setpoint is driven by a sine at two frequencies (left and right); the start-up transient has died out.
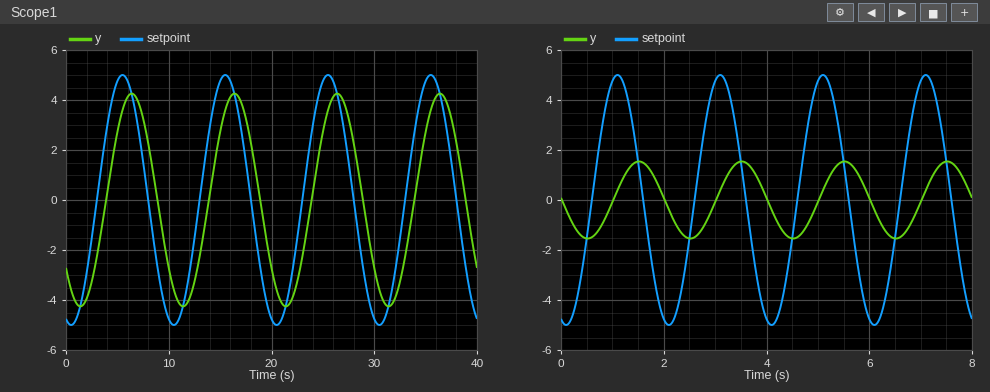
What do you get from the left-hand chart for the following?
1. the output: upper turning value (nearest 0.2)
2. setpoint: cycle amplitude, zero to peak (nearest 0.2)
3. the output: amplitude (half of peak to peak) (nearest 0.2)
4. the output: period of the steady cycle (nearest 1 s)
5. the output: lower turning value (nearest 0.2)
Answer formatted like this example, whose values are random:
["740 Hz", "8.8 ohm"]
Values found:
["4.2", "5.0", "4.2", "10 s", "-4.2"]
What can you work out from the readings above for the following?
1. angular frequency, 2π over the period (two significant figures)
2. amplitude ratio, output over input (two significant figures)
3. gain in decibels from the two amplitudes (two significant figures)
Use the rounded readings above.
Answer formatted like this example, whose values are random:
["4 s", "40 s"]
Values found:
["0.63 rad/s", "0.84", "-1.5 dB"]
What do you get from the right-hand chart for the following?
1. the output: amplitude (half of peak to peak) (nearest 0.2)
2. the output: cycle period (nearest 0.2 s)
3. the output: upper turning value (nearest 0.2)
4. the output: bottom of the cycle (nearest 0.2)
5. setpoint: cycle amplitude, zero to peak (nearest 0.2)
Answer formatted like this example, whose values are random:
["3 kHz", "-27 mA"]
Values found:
["1.6", "2.0 s", "1.6", "-1.6", "5.0"]
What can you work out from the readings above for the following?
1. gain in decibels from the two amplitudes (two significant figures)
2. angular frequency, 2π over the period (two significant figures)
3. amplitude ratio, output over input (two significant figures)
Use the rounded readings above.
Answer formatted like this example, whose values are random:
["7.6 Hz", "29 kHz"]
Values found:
["-9.9 dB", "3.1 rad/s", "0.32"]
